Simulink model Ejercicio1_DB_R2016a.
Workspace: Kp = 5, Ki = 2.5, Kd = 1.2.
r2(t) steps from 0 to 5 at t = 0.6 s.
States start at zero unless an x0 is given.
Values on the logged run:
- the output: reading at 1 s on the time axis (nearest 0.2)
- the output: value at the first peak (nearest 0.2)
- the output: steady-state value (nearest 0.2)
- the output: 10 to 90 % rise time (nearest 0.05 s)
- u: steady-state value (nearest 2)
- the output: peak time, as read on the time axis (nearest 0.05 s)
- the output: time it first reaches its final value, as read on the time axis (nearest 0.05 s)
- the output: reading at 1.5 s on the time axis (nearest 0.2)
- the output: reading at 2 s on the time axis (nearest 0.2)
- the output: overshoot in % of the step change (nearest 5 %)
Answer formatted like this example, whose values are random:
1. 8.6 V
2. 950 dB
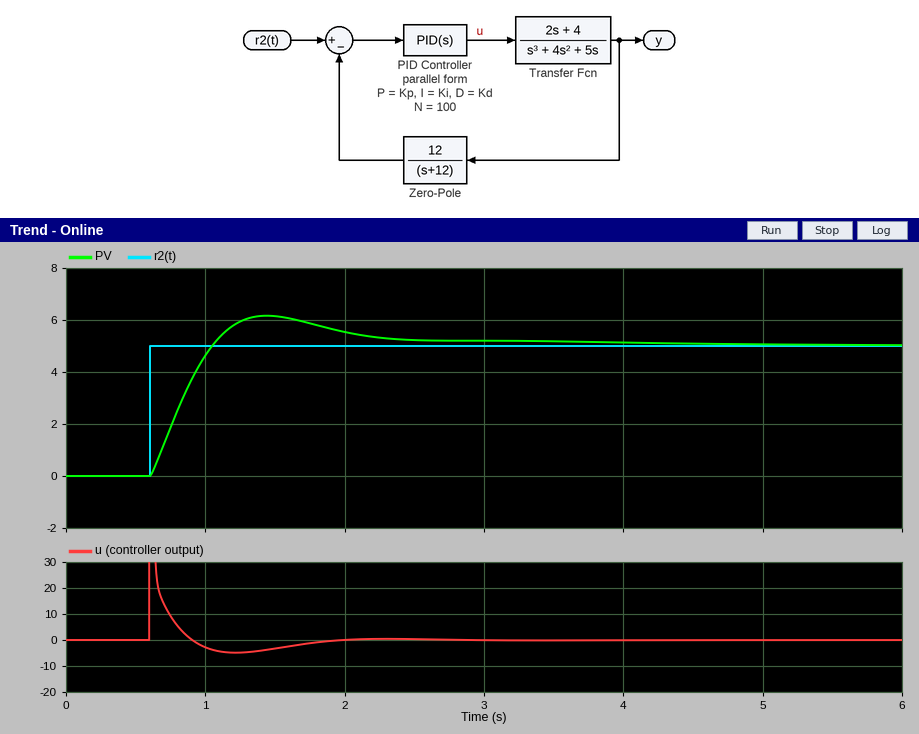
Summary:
1. 4.6
2. 6.2
3. 5.0
4. 0.35 s
5. 0
6. 1.45 s
7. 1.05 s
8. 6.2
9. 5.6
10. 25 %
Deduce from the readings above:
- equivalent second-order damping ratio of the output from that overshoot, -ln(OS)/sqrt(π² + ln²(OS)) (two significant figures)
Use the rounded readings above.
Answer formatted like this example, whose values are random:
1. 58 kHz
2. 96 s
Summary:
1. 0.40
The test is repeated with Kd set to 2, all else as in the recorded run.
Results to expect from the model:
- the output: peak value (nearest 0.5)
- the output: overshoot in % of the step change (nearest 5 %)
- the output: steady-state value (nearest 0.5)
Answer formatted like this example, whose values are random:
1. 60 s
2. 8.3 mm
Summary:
1. 5.5
2. 10 %
3. 5.0
